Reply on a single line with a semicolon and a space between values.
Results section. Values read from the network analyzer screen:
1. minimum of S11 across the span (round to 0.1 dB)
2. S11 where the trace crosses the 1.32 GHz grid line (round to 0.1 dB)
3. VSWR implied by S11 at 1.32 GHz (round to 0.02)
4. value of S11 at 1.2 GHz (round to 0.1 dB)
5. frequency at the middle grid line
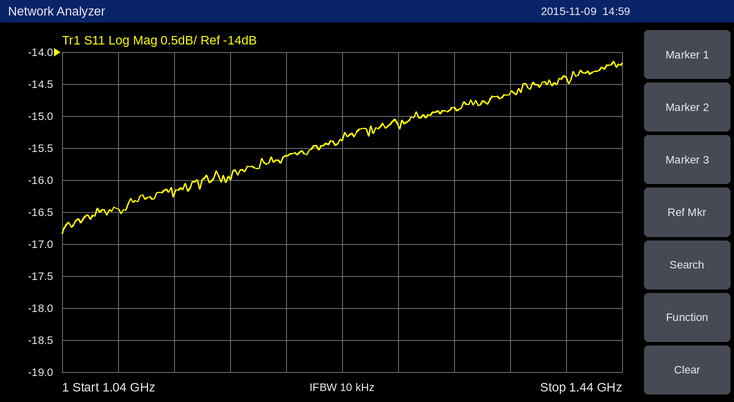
-16.8 dB; -14.9 dB; 1.44; -15.6 dB; 1.24 GHz
